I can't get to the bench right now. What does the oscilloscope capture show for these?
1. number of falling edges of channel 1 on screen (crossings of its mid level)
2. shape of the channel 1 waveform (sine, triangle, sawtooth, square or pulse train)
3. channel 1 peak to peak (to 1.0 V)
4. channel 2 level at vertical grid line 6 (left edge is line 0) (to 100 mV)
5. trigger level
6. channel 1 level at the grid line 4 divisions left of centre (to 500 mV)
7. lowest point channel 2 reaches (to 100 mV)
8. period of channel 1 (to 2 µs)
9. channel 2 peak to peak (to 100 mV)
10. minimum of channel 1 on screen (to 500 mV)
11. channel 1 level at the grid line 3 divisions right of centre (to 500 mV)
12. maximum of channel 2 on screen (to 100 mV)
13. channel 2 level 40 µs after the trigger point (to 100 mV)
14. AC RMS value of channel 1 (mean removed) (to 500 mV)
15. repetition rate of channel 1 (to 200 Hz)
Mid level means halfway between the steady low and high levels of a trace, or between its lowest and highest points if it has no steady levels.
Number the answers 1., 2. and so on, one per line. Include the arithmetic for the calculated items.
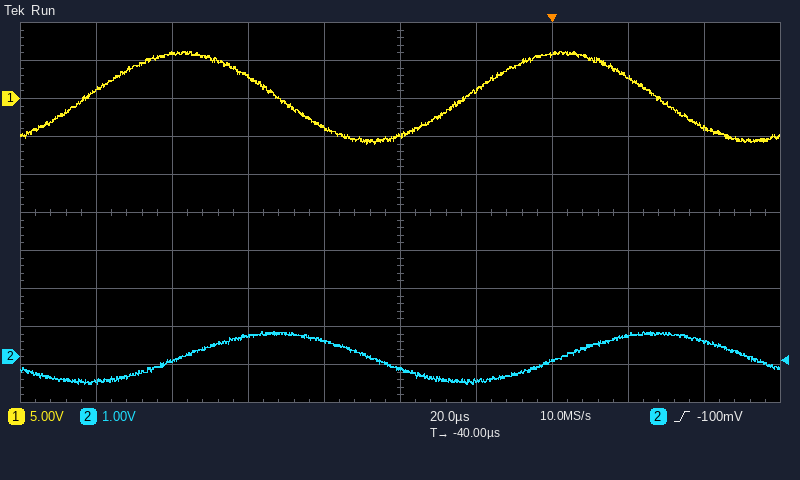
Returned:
1. 2
2. sine
3. 12.0 V
4. -600 mV
5. -100 mV
6. 1.0 V
7. -700 mV
8. 100 µs
9. 700 mV − (-700 mV) = 1.4 V
10. -6.0 V
11. 3.0 V
12. 700 mV
13. 400 mV
14. 12.0 V / (2√2) ≈ 4.24 V, so 4.0 V to the nearest 500 mV
15. 1 / 100 µs ≈ 10.0 kHz
